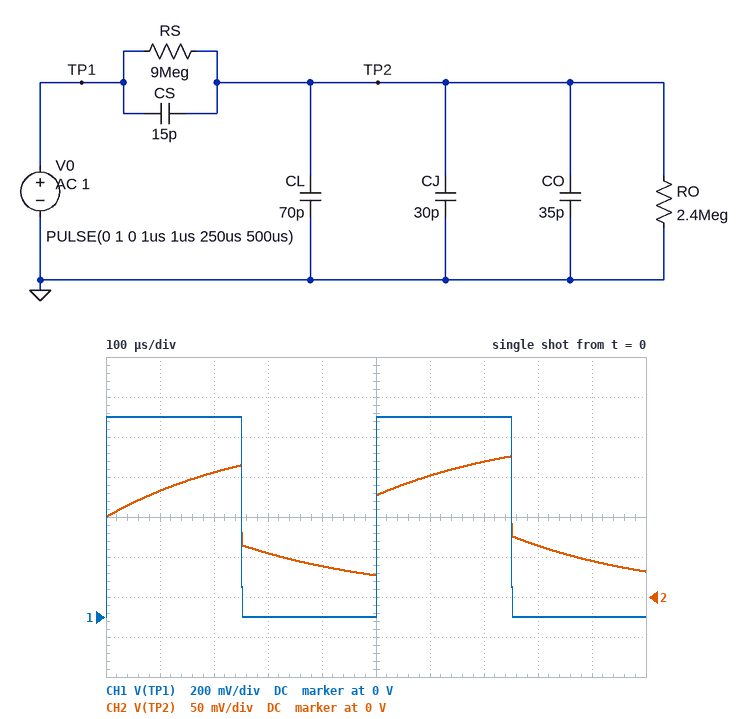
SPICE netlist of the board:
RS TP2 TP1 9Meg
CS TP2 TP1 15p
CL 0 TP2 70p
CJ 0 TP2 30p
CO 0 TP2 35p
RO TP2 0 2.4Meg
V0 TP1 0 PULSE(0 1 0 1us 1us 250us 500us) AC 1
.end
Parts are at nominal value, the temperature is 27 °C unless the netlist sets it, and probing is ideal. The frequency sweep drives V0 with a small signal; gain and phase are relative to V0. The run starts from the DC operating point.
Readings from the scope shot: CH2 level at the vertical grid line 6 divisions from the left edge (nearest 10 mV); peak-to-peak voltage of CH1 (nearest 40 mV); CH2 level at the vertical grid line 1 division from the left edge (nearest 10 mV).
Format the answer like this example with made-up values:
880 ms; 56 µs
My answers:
150 mV; 1.00 V; 130 mV
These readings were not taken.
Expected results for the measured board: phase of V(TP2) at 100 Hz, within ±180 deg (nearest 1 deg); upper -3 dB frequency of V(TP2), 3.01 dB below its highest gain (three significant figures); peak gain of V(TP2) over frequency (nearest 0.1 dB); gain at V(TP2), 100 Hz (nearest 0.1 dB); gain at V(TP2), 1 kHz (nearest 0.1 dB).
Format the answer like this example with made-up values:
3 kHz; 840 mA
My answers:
-5 deg; 756 Hz; -13.5 dB; -13.6 dB; -17.4 dB
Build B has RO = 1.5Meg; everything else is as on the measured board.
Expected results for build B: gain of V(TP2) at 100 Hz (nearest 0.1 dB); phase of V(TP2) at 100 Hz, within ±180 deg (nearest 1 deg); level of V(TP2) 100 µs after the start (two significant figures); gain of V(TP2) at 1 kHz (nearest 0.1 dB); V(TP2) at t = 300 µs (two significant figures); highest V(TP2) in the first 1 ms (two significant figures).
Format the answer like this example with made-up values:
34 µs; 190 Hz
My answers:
-16.9 dB; -2 deg; 120 mV; -18.5 dB; 24 mV; 130 mV
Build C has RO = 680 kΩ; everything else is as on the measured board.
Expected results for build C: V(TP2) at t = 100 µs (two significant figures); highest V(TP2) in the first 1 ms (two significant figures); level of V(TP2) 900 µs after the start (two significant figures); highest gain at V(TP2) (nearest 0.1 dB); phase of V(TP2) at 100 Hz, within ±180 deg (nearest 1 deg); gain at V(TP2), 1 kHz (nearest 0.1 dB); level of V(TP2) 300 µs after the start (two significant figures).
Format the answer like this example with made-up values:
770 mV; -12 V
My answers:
81 mV; 100 mV; -5.8 mV; -20.0 dB; 1 deg; -22.0 dB; -17 mV
